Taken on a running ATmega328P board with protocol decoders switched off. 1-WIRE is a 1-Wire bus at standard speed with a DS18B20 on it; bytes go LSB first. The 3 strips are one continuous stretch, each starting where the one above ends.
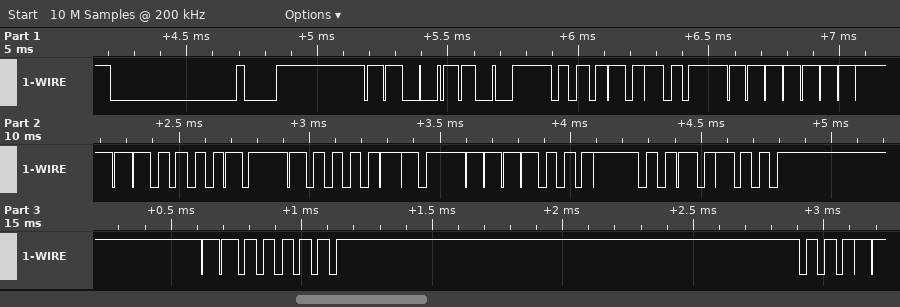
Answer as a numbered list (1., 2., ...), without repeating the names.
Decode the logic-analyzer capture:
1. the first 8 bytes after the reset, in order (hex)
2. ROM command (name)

1. 33 28 FF 43 61 8F 14 03
2. Read ROM
